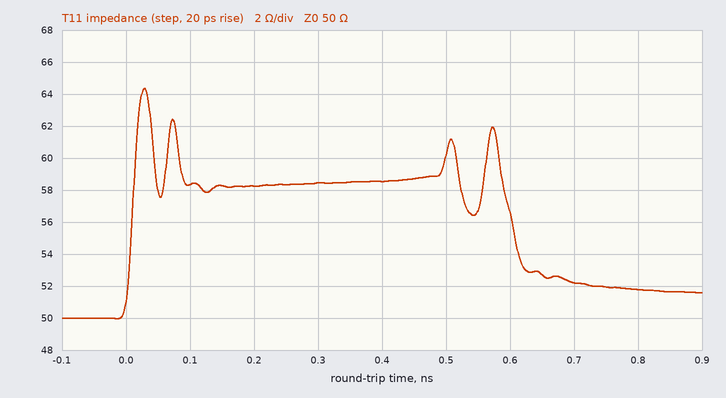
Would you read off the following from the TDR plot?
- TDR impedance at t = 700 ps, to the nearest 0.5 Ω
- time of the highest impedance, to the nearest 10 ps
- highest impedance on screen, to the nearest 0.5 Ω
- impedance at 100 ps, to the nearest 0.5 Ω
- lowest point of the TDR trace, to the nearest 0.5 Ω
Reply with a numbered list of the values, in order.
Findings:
1. 52.0 Ω
2. 30 ps
3. 64.5 Ω
4. 58.5 Ω
5. 50.0 Ω
